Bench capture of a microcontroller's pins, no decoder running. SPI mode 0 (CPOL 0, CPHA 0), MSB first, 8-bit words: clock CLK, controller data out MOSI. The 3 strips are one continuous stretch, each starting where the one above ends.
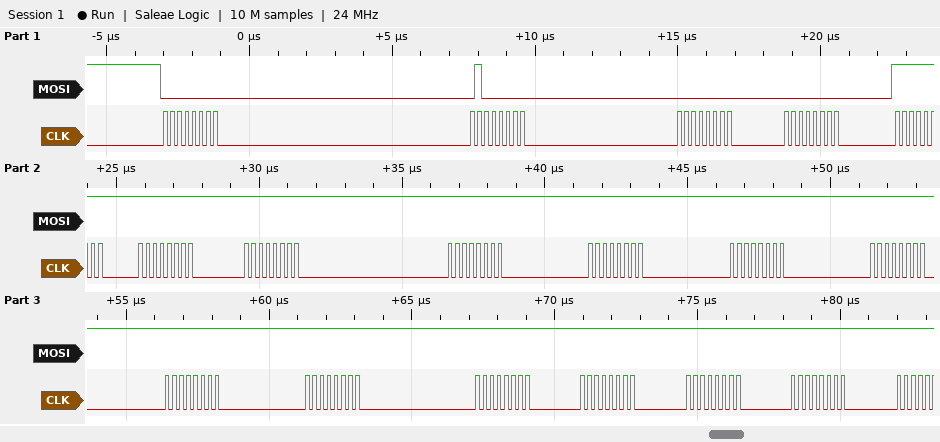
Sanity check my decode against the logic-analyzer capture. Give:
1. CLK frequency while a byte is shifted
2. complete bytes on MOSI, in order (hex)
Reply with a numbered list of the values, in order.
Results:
1. 4 MHz
2. 0x00 0x40 0x00 0x00 0xFF 0xFF 0xFF 0xFF 0xFF 0xFF 0xFF 0xFF 0xFF 0xFF 0xFF 0xFF 0xFF
